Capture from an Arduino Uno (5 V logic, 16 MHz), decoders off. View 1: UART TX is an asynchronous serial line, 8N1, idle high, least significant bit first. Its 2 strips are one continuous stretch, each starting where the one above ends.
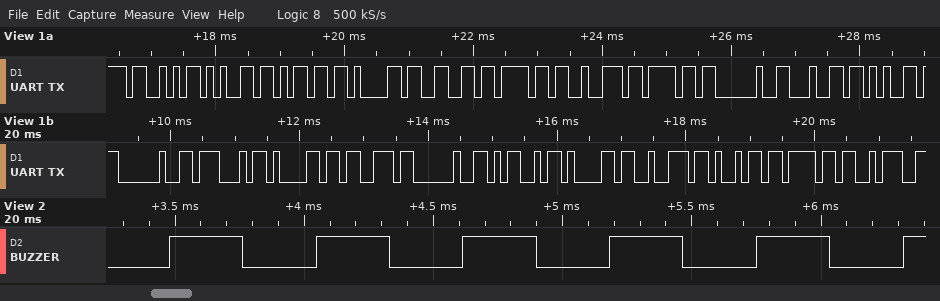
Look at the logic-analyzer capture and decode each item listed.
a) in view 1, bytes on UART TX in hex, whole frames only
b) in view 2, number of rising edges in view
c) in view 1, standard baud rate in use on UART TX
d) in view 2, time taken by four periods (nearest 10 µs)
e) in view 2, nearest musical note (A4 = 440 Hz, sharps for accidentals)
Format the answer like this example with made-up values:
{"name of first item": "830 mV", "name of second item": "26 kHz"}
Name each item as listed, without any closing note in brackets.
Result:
{"in view 1, bytes on UART TX in hex, whole frames only": "53 65 6D 61 66 6F 72 6F 20 64 65 20 47 61 73 20 4D 61 72 69 6F 3A", "in view 2, number of rising edges in view": "6", "in view 1, standard baud rate in use on UART TX": "9600 baud", "in view 2, time taken by four periods": "2270 µs", "in view 2, nearest musical note": "A6"}
